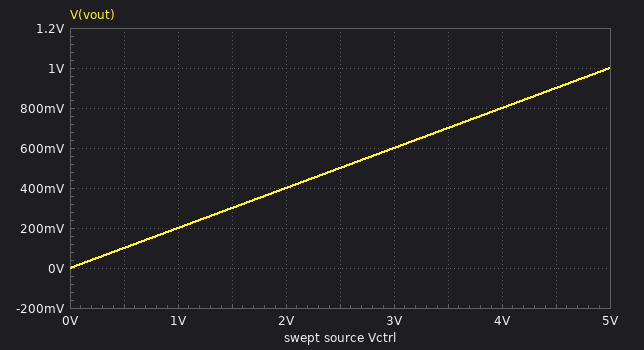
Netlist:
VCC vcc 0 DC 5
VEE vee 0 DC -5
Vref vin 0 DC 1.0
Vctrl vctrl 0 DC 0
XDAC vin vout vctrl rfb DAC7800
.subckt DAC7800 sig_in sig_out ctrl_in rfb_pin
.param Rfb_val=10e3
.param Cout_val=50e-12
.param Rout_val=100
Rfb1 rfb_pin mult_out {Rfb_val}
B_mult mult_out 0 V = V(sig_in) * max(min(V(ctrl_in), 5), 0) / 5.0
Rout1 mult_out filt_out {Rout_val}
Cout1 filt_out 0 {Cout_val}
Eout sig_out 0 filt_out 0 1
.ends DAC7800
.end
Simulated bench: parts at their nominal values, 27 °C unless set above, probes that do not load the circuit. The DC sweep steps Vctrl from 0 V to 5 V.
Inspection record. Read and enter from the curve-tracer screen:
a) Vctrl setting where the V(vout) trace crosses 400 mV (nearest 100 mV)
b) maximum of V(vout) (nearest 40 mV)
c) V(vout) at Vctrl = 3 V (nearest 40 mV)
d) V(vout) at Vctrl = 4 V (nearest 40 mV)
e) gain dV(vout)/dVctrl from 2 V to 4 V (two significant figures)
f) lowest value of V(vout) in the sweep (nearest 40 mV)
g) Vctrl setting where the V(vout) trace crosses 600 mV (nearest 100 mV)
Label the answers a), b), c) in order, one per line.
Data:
a) 2.0 V
b) 1.00 V
c) 600 mV
d) 800 mV
e) 0.20 V/V
f) 0 V
g) 3.0 V
